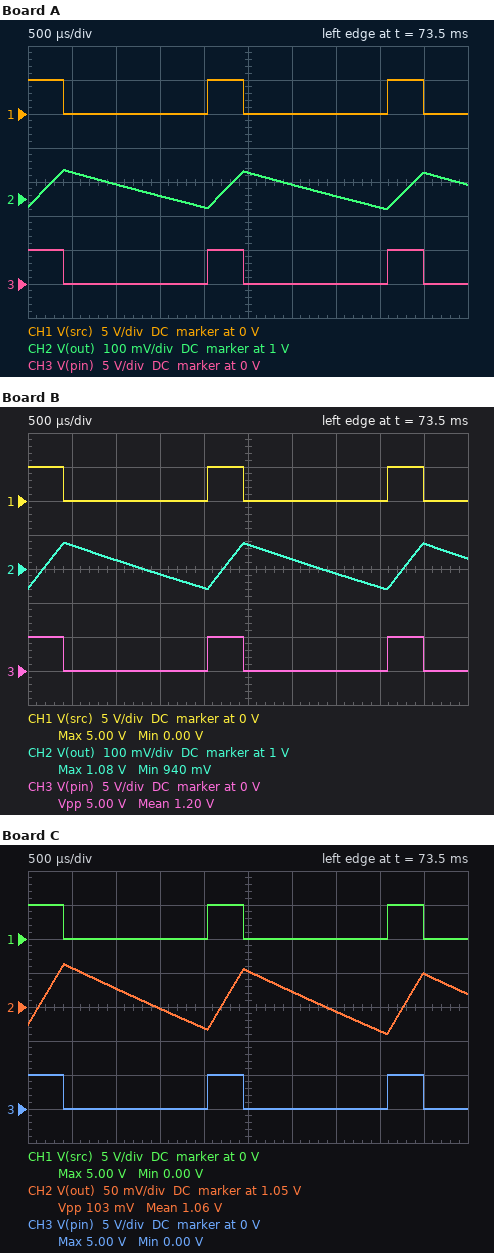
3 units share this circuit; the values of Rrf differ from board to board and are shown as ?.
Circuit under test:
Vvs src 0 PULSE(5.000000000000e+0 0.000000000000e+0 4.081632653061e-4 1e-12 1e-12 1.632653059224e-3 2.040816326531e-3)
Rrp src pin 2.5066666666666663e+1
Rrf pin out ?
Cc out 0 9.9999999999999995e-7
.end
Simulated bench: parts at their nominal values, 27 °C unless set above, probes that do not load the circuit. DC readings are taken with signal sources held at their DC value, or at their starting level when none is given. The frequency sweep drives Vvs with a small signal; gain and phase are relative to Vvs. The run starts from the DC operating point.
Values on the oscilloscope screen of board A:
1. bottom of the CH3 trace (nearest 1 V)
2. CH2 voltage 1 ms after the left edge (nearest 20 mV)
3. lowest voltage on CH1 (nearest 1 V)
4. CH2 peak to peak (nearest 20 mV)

0 V
1.04 V
0 V
120 mV
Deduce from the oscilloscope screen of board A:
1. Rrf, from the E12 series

15 kΩ
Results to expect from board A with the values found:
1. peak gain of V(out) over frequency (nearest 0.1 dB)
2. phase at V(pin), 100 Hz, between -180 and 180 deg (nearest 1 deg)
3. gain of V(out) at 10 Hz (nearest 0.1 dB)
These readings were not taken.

0 dB
0 deg
-2.8 dB
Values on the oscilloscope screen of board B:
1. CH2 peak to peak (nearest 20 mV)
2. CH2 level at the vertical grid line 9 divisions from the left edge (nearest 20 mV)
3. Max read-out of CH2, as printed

140 mV
1.08 V
1.08 V
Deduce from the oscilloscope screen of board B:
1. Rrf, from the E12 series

12 kΩ
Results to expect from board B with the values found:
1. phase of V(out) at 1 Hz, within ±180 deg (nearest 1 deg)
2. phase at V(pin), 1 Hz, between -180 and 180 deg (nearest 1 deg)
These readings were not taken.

-4 deg
0 deg
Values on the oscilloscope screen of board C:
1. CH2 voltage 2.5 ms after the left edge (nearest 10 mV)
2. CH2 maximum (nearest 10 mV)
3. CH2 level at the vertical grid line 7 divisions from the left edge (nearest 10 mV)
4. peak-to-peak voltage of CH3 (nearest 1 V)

1.10 V
1.11 V
1.04 V
5 V
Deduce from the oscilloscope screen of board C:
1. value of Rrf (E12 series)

18 kΩ
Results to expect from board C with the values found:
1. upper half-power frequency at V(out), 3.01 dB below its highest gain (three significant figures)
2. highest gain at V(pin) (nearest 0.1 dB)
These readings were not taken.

8.83 Hz
0 dB
